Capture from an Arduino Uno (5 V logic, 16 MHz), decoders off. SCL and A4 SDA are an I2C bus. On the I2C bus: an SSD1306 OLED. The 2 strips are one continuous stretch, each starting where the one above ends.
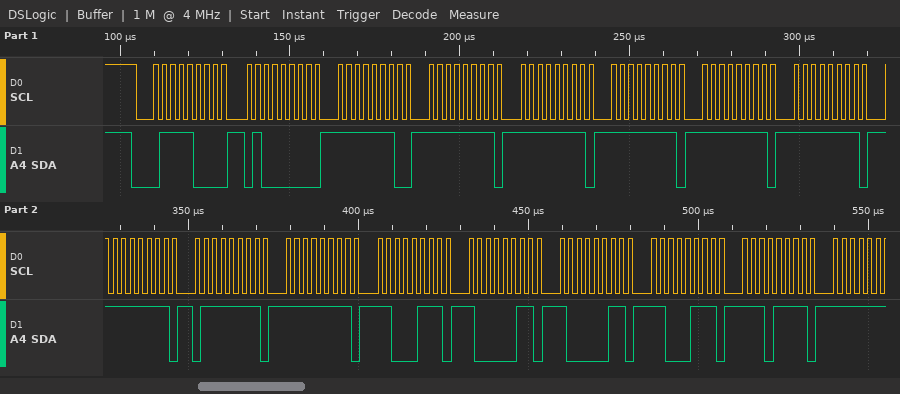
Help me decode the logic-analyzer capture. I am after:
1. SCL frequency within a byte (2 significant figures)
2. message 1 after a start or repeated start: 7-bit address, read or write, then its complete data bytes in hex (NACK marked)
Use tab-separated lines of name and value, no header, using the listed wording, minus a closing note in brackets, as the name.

SCL frequency within a byte	400 kHz
message 1 after a start or repeated start: 7-bit address, read or write, then its complete data bytes in hex	0x3C write: 40 FE FF FF FF FF FF FF 7F FF C7 83 83 C7 EF
